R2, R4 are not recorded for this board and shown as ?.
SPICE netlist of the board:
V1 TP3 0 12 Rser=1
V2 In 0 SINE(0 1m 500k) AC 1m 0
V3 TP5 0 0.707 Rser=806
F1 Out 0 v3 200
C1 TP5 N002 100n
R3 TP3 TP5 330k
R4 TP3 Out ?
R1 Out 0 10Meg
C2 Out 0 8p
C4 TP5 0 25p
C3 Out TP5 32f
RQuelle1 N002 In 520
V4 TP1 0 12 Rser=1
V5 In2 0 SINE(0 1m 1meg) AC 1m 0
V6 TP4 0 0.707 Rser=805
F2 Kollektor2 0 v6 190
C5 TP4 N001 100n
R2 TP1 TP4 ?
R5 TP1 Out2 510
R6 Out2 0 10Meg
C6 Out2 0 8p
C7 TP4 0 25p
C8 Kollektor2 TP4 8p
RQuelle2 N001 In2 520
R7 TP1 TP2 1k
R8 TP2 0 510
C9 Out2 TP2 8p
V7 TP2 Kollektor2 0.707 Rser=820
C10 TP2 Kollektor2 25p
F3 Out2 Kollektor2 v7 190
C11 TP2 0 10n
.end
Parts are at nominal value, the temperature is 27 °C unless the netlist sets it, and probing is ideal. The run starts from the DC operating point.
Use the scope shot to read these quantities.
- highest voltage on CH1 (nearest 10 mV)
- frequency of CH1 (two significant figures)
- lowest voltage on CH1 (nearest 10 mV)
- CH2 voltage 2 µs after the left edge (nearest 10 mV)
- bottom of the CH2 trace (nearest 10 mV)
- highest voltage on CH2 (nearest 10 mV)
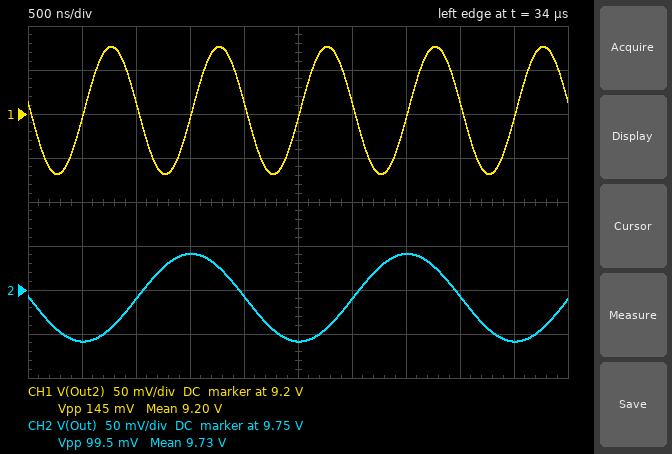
9.28 V
1.0 MHz
9.13 V
9.74 V
9.69 V
9.79 V
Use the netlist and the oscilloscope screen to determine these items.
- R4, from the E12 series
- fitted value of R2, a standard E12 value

330 Ω
390 kΩ
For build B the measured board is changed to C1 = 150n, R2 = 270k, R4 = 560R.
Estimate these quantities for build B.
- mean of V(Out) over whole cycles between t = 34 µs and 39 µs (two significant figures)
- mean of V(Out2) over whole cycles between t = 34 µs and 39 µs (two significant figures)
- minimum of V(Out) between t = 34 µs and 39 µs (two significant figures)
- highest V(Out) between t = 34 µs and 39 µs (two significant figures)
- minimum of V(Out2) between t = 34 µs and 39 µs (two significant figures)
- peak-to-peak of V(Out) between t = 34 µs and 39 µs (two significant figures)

8.2 V
8.0 V
8.1 V
8.3 V
7.9 V
170 mV
